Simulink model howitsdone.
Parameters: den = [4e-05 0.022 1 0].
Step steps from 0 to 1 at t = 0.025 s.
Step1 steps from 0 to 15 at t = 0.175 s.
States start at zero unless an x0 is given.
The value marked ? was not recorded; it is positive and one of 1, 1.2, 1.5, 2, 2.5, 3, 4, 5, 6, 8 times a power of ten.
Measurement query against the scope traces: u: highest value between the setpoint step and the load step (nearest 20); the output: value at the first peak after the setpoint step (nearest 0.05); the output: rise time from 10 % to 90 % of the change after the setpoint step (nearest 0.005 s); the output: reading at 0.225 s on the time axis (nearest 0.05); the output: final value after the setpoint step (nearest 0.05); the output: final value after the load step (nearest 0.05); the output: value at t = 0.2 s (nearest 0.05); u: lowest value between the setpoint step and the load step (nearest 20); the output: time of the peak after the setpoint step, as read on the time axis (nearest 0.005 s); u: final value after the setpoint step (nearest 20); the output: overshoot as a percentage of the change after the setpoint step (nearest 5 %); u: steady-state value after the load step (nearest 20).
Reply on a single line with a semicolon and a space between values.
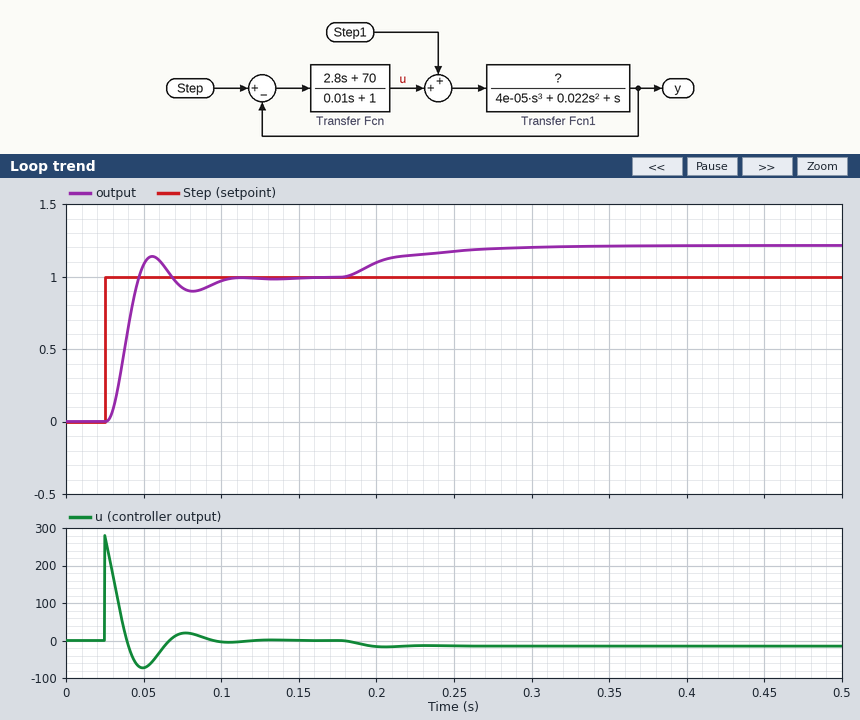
280; 1.15; 0.015 s; 1.15; 1.00; 1.20; 1.10; -80; 0.055 s; 0; 15 %; -20
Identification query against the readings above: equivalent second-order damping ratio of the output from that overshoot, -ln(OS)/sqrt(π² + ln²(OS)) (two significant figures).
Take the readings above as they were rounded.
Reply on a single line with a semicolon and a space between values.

0.52
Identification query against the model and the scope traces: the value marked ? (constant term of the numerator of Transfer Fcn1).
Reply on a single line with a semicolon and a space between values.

1
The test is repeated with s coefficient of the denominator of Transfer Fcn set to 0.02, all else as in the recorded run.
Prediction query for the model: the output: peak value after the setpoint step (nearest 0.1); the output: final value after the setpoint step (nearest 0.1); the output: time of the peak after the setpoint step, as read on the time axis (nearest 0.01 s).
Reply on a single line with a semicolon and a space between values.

1.2; 1.0; 0.07 s
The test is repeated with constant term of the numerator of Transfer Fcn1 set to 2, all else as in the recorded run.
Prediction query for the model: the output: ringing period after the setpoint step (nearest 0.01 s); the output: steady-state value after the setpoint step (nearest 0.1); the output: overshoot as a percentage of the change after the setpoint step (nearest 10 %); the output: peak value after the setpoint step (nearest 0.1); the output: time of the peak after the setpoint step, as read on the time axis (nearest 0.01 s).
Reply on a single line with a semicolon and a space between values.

0.04 s; 1.0; 40 %; 1.4; 0.05 s
